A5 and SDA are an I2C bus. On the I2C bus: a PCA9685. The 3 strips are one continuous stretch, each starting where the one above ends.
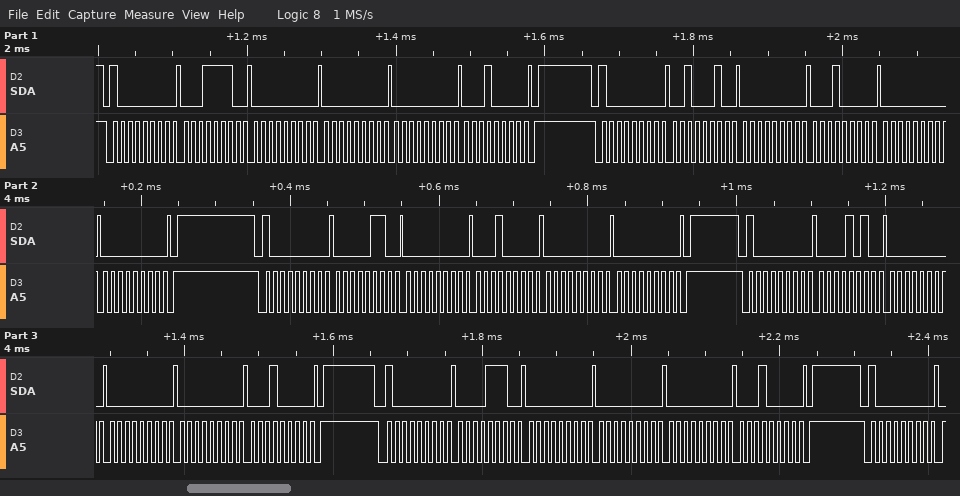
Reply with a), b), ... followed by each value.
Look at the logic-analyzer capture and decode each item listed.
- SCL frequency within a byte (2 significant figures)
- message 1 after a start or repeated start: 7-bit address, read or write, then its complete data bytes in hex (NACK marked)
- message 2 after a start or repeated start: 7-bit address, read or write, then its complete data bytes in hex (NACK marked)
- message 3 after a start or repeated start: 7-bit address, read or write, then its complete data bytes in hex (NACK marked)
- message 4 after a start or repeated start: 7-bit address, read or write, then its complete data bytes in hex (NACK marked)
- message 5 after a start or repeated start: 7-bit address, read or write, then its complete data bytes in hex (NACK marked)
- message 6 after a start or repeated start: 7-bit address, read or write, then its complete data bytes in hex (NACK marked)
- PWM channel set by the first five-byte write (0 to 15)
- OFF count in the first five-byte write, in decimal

a) 100 kHz
b) 0x40 write: 1E 00 00 00 10
c) 0x40 write: 22 00 10 00 00
d) 0x40 write: 06 00 10 00 00
e) 0x40 write: 0A 00 00 00 10
f) 0x40 write: 0E 00 00 00 10
g) 0x40 write
h) 6
i) 4096
